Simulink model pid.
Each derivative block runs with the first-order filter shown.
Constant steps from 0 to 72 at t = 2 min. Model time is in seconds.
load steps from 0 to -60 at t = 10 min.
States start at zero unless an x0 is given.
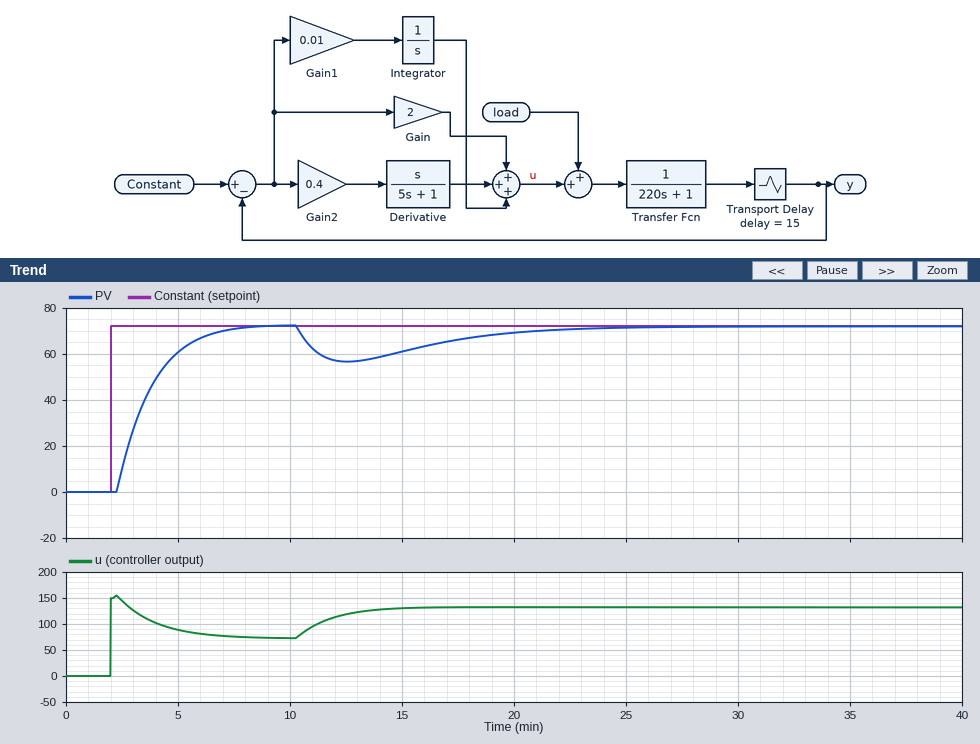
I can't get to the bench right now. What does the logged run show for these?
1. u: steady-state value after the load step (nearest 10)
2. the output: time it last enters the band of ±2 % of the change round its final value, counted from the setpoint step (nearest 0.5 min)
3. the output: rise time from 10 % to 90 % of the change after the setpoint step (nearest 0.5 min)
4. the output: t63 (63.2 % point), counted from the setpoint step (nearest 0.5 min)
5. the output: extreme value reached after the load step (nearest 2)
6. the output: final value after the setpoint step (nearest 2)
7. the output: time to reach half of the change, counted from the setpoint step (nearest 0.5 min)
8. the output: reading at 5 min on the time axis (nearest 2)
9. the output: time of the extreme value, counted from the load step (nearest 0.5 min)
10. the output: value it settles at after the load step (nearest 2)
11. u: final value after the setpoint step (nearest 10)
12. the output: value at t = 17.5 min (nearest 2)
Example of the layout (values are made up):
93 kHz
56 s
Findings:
130
5.5 min
3.0 min
2.0 min
56
72
1.5 min
60
2.5 min
72
70
66
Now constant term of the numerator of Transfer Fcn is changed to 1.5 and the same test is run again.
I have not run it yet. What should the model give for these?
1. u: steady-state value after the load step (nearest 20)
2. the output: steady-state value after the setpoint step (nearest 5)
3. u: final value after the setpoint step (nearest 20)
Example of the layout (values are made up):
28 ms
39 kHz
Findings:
100
70
40
